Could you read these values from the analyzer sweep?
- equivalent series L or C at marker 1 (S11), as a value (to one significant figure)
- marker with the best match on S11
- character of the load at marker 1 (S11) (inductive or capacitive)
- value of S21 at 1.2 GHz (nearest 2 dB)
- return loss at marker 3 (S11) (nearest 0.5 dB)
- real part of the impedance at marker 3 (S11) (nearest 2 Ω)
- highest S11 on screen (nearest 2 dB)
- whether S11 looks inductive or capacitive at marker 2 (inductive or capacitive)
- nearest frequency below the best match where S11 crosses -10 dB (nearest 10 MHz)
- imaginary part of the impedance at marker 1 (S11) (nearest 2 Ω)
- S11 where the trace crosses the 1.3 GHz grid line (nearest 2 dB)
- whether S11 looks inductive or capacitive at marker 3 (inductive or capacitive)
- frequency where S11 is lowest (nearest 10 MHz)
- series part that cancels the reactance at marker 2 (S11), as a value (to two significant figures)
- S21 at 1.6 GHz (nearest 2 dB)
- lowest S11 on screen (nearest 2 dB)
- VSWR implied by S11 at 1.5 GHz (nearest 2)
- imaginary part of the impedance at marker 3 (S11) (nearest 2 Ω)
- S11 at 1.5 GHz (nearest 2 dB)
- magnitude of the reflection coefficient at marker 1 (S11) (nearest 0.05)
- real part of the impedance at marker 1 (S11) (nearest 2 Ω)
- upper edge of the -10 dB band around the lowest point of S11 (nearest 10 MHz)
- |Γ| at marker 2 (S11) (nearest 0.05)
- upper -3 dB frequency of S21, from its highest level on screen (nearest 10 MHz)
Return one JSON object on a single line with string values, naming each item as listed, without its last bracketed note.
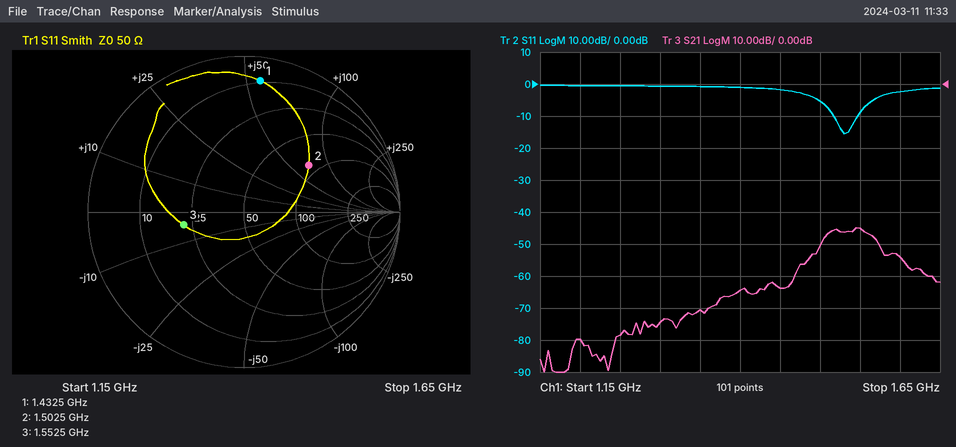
{"equivalent series L or C at marker 1 (S11), as a value": "6 nH", "marker with the best match on S11": "marker 3", "character of the load at marker 1 (S11)": "inductive", "value of S21 at 1.2 GHz": "-80 dB", "return loss at marker 3 (S11)": "8.0 dB", "real part of the impedance at marker 3 (S11)": "22 Ω", "highest S11 on screen": "0 dB", "whether S11 looks inductive or capacitive at marker 2": "inductive", "nearest frequency below the best match where S11 crosses -10 dB": "1.52 GHz", "imaginary part of the impedance at marker 1 (S11)": "+56 Ω", "S11 where the trace crosses the 1.3 GHz grid line": "0 dB", "whether S11 looks inductive or capacitive at marker 3": "capacitive", "frequency where S11 is lowest": "1.53 GHz", "series part that cancels the reactance at marker 2 (S11), as a value": "1.5 pF", "S21 at 1.6 GHz": "-54 dB", "lowest S11 on screen": "-16 dB", "VSWR implied by S11 at 1.5 GHz": "4", "imaginary part of the impedance at marker 3 (S11)": "-4 Ω", "S11 at 1.5 GHz": "-6 dB", "magnitude of the reflection coefficient at marker 1 (S11)": "0.85", "real part of the impedance at marker 1 (S11)": "10 Ω", "upper edge of the -10 dB band around the lowest point of S11": "1.55 GHz", "|Γ| at marker 2 (S11)": "0.50", "upper -3 dB frequency of S21, from its highest level on screen": "1.57 GHz"}
